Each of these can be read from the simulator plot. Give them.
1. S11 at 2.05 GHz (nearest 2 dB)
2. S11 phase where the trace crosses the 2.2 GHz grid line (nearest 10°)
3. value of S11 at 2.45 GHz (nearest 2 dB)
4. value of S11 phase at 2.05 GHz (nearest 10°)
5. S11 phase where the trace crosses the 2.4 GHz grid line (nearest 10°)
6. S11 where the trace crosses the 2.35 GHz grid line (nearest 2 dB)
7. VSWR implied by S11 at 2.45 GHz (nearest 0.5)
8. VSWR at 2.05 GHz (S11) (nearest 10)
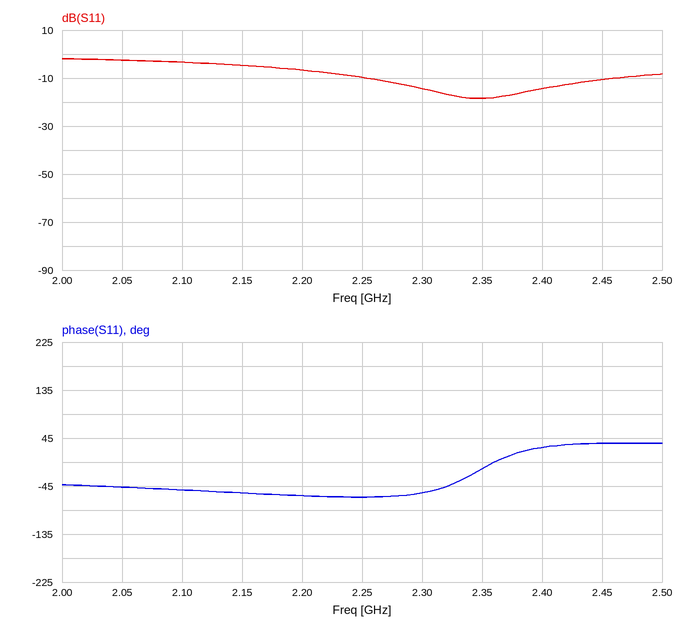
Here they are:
-2 dB
-60°
-10 dB
-50°
30°
-18 dB
2.0
10
